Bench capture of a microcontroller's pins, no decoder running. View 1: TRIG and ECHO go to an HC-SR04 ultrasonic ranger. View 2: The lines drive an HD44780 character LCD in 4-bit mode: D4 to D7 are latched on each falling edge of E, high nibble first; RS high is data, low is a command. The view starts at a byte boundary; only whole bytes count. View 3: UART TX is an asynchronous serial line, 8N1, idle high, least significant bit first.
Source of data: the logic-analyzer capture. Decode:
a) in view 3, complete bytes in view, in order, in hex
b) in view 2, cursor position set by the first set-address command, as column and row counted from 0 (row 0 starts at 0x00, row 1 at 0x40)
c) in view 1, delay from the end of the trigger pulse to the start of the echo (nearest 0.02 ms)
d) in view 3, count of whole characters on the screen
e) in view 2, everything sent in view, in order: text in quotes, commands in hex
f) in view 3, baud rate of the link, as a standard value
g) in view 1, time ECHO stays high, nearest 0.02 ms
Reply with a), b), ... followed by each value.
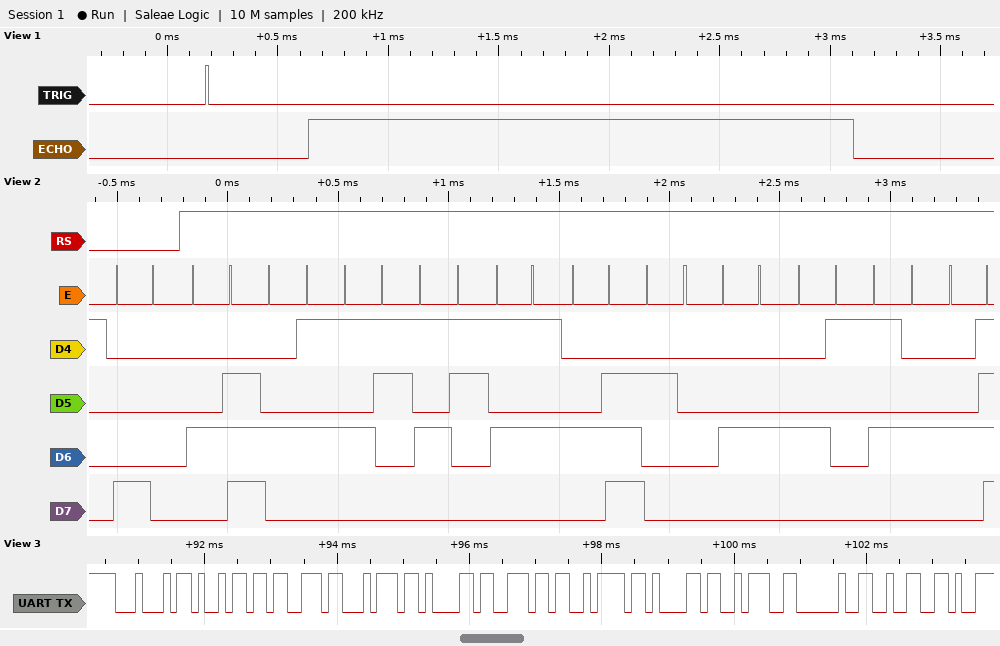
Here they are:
a) 44 69 73 74 61 6E 7A 61 3A 20 32
b) column 0, row 0
c) 0.46 ms
d) 11
e) 0x80 "NESSUN DATO"
f) 9600 baud
g) 2.46 ms
